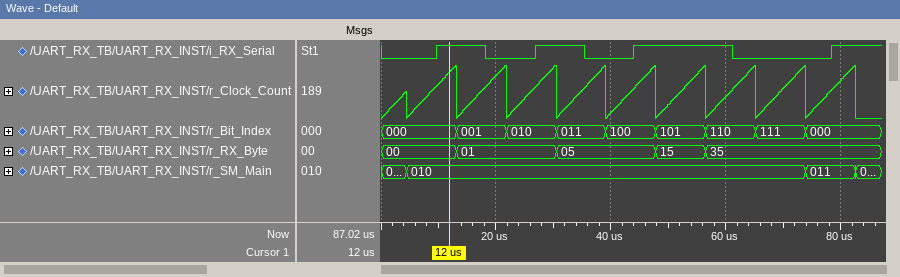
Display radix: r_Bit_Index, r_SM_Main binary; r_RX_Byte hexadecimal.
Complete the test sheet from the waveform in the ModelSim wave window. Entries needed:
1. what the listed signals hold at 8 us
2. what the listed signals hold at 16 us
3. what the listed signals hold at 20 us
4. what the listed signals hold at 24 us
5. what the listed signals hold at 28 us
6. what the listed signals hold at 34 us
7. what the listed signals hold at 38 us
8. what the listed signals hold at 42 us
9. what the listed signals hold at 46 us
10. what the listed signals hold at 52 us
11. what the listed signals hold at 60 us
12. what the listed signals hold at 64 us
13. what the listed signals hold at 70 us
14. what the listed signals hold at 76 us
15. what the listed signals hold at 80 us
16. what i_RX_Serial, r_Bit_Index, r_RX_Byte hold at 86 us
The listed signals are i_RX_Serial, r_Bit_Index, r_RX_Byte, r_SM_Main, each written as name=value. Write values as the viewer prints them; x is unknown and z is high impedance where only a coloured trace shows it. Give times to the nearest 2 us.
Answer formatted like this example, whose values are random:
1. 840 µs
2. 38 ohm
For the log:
1. i_RX_Serial=0, r_Bit_Index=000, r_RX_Byte=00, r_SM_Main=010
2. i_RX_Serial=1, r_Bit_Index=001, r_RX_Byte=01, r_SM_Main=010
3. i_RX_Serial=0, r_Bit_Index=001, r_RX_Byte=01, r_SM_Main=010
4. i_RX_Serial=0, r_Bit_Index=010, r_RX_Byte=01, r_SM_Main=010
5. i_RX_Serial=1, r_Bit_Index=010, r_RX_Byte=01, r_SM_Main=010
6. i_RX_Serial=1, r_Bit_Index=011, r_RX_Byte=05, r_SM_Main=010
7. i_RX_Serial=0, r_Bit_Index=011, r_RX_Byte=05, r_SM_Main=010
8. i_RX_Serial=0, r_Bit_Index=100, r_RX_Byte=05, r_SM_Main=010
9. i_RX_Serial=1, r_Bit_Index=100, r_RX_Byte=05, r_SM_Main=010
10. i_RX_Serial=1, r_Bit_Index=101, r_RX_Byte=15, r_SM_Main=010
11. i_RX_Serial=1, r_Bit_Index=110, r_RX_Byte=35, r_SM_Main=010
12. i_RX_Serial=0, r_Bit_Index=110, r_RX_Byte=35, r_SM_Main=010
13. i_RX_Serial=0, r_Bit_Index=111, r_RX_Byte=35, r_SM_Main=010
14. i_RX_Serial=0, r_Bit_Index=000, r_RX_Byte=35, r_SM_Main=011
15. i_RX_Serial=1, r_Bit_Index=000, r_RX_Byte=35, r_SM_Main=011
16. i_RX_Serial=1, r_Bit_Index=000, r_RX_Byte=35
